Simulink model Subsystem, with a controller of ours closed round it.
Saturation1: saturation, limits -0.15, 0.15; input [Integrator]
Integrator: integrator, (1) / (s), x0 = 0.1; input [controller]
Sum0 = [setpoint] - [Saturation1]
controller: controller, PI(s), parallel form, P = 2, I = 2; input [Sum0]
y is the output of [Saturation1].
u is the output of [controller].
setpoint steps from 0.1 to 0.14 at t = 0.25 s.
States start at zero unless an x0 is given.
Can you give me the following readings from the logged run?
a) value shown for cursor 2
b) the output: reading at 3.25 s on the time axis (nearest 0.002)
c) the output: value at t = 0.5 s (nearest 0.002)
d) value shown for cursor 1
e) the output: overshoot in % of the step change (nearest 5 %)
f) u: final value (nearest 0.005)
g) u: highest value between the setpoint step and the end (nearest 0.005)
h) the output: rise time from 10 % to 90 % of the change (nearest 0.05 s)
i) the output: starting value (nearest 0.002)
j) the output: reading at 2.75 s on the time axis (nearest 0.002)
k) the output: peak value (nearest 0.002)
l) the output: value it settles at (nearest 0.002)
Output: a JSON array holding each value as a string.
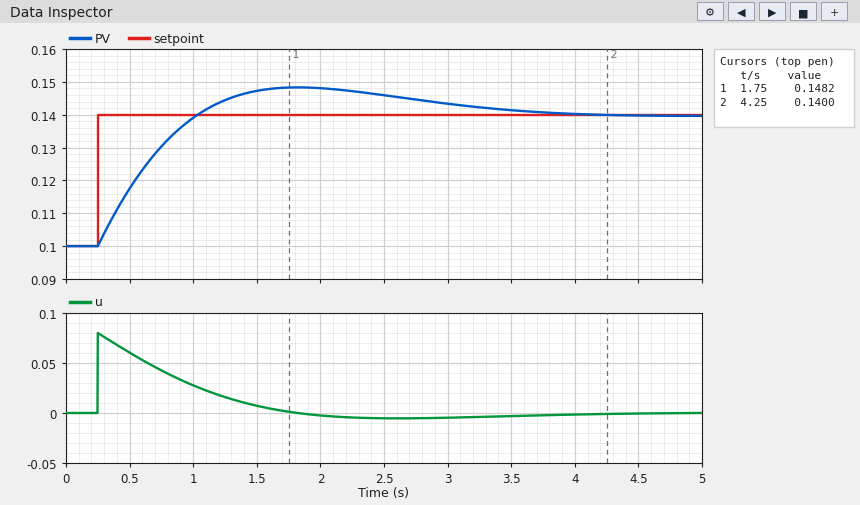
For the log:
["0.1400", "0.142", "0.118", "0.1482", "20 %", "0.000", "0.080", "0.60 s", "0.100", "0.144", "0.148", "0.140"]
